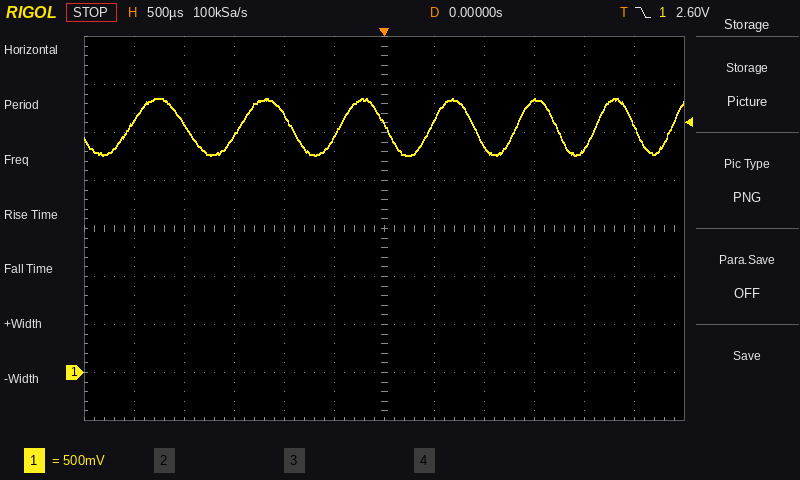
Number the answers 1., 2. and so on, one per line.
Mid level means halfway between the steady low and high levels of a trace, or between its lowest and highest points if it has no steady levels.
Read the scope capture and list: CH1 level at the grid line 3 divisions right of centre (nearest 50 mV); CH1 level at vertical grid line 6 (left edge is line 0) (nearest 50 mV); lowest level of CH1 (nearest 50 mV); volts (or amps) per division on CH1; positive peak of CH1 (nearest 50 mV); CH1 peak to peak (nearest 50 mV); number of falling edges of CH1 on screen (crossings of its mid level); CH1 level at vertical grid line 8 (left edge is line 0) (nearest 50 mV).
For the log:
1. 2.85 V
2. 2.60 V
3. 2.25 V
4. 500 mV
5. 2.85 V
6. 600 mV
7. 6
8. 2.35 V
